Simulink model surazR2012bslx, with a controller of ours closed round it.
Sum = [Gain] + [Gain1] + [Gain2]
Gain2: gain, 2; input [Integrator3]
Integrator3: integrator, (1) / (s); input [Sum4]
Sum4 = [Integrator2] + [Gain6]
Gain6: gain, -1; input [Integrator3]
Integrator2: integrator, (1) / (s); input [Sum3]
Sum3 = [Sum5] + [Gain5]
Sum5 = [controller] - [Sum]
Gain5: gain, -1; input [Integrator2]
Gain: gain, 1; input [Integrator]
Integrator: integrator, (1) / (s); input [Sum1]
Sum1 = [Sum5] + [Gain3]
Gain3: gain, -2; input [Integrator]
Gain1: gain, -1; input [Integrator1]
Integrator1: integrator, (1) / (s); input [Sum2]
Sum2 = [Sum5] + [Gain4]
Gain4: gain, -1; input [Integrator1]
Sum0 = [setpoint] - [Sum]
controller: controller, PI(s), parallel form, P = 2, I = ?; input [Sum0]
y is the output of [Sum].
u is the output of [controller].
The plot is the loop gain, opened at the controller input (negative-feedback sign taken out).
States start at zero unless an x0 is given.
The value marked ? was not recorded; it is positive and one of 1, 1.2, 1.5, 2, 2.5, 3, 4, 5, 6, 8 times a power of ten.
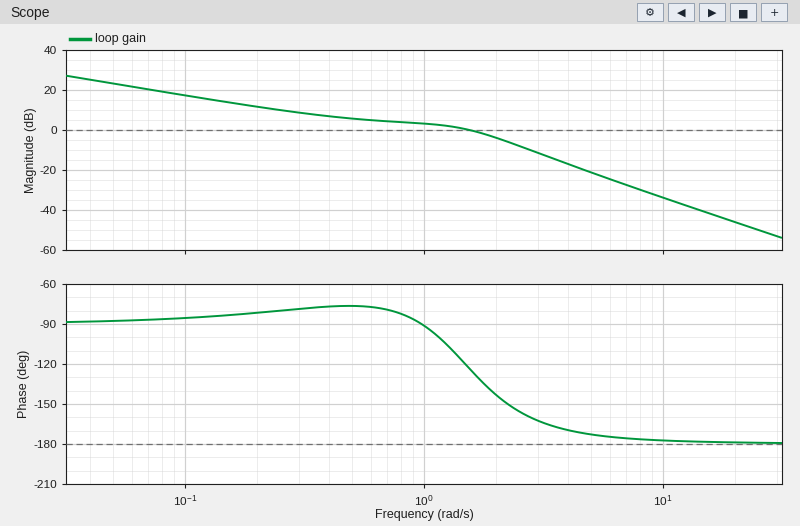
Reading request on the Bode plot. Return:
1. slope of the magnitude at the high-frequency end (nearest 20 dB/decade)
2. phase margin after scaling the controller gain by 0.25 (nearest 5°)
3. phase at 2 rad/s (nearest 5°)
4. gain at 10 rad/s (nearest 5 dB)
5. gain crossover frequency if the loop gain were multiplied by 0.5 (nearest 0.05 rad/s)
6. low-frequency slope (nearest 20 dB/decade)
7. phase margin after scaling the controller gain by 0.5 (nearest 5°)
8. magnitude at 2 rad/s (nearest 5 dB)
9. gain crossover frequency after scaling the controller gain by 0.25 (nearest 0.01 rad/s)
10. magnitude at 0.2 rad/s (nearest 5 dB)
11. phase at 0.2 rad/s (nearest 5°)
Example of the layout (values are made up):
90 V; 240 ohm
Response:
-40 dB/decade; 100°; -145°; -35 dB; 0.45 rad/s; -20 dB/decade; 105°; -5 dB; 0.19 rad/s; 10 dB; -80°
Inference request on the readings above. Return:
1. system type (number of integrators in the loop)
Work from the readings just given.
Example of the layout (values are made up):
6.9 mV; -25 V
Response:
1
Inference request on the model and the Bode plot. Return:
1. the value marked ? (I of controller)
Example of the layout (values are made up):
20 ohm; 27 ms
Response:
1.2
